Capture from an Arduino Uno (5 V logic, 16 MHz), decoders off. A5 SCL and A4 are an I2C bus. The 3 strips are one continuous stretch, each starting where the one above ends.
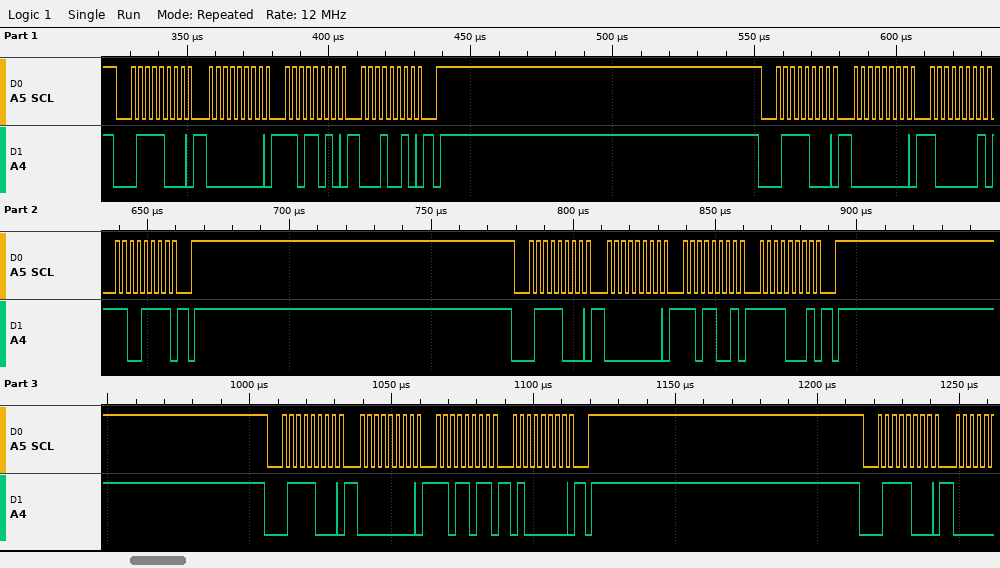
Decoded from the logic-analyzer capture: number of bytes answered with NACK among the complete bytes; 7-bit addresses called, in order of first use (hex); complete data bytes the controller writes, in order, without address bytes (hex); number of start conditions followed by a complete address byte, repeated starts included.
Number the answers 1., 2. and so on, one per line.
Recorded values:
1. 0
2. 0x3C
3. 00 DA 12 00 81 CF 00 D9 F1 00 DB 40
4. 5
